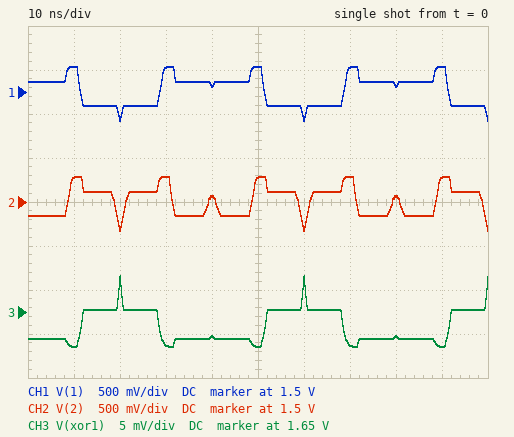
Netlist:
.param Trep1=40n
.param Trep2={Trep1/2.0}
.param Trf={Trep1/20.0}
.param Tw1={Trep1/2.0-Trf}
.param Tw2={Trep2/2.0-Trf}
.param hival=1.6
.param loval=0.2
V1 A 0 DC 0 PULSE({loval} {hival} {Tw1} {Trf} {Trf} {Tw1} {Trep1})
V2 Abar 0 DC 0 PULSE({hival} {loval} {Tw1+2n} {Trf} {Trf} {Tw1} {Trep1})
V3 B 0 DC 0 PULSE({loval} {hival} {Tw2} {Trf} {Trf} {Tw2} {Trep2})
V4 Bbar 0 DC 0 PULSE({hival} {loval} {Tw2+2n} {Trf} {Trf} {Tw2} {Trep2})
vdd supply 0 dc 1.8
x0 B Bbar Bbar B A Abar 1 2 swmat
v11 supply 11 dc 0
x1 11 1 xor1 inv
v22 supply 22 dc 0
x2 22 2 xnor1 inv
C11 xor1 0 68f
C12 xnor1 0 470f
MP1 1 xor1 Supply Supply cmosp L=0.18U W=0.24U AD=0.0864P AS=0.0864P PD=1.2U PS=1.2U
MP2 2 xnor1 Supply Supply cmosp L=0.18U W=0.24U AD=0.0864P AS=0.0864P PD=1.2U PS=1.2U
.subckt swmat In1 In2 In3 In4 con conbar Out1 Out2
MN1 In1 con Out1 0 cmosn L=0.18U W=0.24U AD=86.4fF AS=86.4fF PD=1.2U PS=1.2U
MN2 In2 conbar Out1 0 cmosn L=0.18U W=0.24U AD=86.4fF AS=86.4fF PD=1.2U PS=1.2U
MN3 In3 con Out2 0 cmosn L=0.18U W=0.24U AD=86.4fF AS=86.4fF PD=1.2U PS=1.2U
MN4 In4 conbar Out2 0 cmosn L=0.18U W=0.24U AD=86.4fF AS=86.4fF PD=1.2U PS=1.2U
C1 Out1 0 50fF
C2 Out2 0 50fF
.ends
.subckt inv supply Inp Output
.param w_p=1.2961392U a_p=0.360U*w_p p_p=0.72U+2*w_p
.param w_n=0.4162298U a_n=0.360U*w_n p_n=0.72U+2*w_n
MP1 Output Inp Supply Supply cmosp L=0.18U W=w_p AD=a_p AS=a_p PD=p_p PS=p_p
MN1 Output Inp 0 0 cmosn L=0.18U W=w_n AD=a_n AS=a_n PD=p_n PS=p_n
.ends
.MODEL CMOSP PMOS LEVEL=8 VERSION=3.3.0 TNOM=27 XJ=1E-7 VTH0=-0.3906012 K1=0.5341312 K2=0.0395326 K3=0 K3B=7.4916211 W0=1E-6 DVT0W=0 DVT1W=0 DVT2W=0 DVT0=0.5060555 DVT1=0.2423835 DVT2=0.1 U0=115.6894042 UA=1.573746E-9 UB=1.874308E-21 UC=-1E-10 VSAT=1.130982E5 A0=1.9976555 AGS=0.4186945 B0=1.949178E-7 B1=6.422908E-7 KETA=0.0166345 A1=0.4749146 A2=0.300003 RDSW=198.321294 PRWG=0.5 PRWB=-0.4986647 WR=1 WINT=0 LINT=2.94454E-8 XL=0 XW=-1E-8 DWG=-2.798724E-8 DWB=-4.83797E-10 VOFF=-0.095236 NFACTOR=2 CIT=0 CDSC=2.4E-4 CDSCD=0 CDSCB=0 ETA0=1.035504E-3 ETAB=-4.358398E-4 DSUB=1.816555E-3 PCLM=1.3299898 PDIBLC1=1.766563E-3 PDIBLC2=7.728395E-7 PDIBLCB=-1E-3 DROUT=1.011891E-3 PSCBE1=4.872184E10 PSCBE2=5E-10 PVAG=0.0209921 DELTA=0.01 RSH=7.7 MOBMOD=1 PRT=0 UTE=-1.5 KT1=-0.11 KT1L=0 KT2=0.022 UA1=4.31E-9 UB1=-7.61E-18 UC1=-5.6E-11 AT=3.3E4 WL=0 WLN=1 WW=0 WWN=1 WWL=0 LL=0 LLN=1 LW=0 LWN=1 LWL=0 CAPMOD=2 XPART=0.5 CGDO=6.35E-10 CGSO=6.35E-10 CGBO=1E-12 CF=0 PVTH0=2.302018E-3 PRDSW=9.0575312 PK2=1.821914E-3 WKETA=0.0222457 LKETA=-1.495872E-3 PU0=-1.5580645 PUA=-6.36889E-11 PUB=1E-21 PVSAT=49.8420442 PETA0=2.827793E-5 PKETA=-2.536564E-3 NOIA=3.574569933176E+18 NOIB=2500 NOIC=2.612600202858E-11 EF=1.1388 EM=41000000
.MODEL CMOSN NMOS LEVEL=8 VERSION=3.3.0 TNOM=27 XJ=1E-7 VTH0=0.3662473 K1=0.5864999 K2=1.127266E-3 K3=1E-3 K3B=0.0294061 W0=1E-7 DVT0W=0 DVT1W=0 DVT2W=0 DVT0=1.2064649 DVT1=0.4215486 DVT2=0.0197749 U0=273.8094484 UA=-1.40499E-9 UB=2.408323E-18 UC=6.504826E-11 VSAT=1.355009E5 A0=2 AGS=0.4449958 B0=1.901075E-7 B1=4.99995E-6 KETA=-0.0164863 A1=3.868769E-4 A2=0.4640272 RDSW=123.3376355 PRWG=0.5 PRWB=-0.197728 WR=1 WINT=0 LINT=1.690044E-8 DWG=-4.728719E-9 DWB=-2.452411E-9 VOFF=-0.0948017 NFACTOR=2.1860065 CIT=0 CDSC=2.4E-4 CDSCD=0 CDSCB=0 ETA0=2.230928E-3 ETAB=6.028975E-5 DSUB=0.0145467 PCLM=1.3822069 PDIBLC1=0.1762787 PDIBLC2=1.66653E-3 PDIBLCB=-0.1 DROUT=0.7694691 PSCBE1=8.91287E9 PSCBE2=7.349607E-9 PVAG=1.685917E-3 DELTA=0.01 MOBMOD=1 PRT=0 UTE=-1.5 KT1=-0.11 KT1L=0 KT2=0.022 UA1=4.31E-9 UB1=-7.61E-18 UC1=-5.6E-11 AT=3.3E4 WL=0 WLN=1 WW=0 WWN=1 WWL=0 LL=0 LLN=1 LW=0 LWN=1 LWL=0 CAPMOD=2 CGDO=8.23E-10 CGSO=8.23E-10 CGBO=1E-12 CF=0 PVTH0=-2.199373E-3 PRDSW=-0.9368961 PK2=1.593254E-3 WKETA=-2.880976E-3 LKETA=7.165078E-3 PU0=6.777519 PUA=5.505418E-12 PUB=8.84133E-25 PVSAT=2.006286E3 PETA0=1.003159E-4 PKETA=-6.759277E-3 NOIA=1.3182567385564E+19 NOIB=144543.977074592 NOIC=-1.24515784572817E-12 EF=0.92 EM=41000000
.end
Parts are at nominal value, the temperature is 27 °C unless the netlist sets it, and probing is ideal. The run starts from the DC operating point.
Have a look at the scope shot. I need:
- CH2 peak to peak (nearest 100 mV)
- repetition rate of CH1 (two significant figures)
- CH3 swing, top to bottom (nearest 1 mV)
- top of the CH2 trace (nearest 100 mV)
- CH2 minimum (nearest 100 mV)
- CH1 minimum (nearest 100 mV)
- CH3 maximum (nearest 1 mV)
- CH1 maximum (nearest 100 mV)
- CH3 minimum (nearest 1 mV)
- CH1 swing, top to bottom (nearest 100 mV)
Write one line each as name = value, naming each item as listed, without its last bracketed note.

CH2 peak to peak = 600 mV
repetition rate of CH1 = 25 MHz
CH3 swing, top to bottom = 8 mV
top of the CH2 trace = 1.8 V
CH2 minimum = 1.2 V
CH1 minimum = 1.2 V
CH3 maximum = 1.654 V
CH1 maximum = 1.8 V
CH3 minimum = 1.646 V
CH1 swing, top to bottom = 600 mV
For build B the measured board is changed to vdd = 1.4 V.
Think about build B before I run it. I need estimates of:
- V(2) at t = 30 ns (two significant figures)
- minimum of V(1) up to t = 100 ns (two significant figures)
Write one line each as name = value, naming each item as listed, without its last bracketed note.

V(2) at t = 30 ns = 1.4 V
minimum of V(1) up to t = 100 ns = 870 mV
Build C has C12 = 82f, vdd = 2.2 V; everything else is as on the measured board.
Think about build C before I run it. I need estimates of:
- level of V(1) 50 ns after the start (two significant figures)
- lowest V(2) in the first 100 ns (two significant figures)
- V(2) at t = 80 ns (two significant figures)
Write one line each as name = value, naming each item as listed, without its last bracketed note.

level of V(1) 50 ns after the start = 2.2 V
lowest V(2) in the first 100 ns = 1.5 V
V(2) at t = 80 ns = 1.9 V
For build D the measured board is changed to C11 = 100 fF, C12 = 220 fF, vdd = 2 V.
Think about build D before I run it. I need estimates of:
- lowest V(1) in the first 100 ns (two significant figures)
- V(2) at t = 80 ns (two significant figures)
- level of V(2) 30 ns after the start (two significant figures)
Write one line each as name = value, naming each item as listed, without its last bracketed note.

lowest V(1) in the first 100 ns = 1.3 V
V(2) at t = 80 ns = 1.7 V
level of V(2) 30 ns after the start = 2.0 V
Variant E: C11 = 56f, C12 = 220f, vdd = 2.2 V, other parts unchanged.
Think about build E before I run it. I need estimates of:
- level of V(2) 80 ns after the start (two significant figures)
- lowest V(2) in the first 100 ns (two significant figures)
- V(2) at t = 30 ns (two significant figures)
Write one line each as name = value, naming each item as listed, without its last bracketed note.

level of V(2) 80 ns after the start = 1.9 V
lowest V(2) in the first 100 ns = 1.5 V
V(2) at t = 30 ns = 2.2 V
